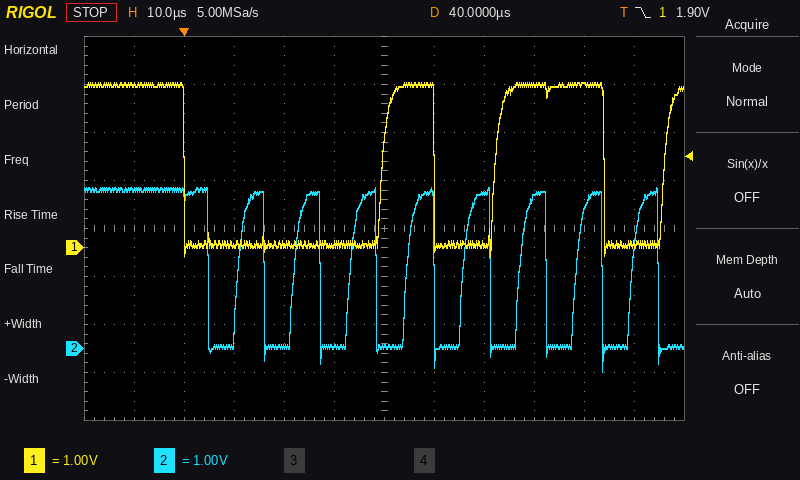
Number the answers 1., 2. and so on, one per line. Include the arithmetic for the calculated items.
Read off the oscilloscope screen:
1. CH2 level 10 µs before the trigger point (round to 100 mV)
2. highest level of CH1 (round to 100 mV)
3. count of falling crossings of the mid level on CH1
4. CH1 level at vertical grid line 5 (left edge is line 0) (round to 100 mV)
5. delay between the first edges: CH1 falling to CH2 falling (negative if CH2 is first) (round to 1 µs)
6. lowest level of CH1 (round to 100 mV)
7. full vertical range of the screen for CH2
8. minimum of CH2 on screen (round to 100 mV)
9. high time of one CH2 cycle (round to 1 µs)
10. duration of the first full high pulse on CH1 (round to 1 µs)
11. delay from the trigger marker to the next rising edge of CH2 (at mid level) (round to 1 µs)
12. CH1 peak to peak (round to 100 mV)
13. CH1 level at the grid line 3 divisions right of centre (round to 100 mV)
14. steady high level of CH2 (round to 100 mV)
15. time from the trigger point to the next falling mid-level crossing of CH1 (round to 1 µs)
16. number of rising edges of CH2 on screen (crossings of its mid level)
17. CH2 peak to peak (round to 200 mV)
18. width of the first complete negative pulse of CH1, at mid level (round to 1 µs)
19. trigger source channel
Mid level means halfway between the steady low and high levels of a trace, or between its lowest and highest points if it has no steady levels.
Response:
1. 3.3 V
2. 3.4 V
3. 3
4. 100 mV
5. +5 µs
6. -200 mV
7. 8 V
8. -500 mV
9. 5 µs
10. 10 µs
11. 11 µs
12. 3.4 V − (-200 mV) = 3.6 V
13. 3.4 V
14. 3.3 V
15. 50 µs
16. 8
17. 3.8 V
18. 40 µs
19. CH1
